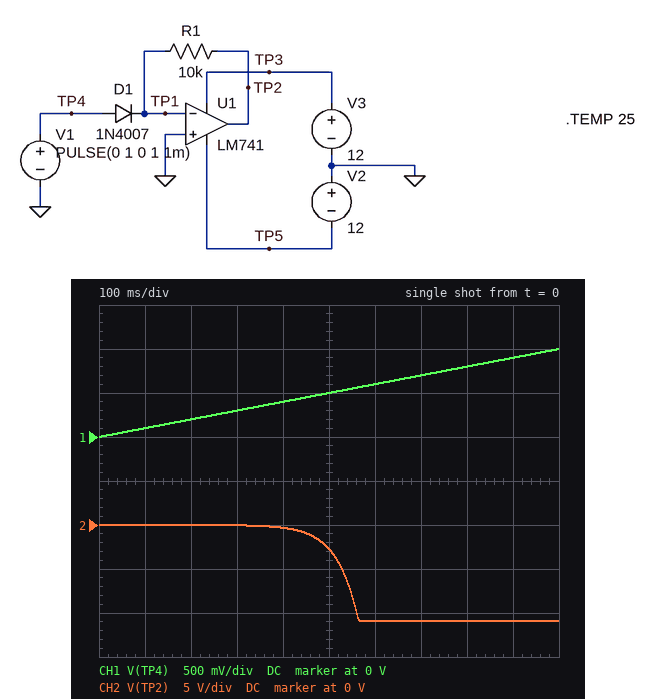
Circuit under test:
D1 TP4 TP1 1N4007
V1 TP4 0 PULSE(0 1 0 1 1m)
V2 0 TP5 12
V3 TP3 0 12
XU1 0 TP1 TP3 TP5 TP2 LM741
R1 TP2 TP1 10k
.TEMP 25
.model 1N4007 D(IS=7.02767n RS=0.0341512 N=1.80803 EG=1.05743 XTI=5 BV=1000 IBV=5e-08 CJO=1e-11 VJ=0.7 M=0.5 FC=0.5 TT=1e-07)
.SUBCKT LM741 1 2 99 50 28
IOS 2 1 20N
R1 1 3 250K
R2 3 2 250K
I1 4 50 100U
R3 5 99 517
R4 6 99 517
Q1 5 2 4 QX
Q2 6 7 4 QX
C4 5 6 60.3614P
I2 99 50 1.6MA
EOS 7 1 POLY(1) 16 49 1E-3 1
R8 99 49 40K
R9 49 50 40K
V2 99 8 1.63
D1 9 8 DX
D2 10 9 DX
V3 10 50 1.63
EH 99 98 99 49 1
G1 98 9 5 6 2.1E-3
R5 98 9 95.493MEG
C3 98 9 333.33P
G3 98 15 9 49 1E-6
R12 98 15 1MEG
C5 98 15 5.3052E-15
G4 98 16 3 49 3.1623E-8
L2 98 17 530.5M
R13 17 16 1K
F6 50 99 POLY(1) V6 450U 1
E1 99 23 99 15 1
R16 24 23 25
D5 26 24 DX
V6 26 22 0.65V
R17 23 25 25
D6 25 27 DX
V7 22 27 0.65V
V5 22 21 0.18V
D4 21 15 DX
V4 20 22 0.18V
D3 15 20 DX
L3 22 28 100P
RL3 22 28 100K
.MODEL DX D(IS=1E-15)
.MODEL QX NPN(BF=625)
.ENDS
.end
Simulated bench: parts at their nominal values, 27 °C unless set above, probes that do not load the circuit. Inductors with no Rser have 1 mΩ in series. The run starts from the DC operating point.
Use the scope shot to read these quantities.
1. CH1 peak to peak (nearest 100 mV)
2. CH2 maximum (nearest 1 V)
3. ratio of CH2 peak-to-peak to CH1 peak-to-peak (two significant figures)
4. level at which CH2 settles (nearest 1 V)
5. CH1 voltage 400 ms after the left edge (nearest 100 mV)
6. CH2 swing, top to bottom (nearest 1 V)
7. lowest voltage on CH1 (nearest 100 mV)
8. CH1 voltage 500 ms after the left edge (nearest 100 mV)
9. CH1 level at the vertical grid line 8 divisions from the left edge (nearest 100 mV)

1.0 V
0 V
11
-11 V
400 mV
11 V
0 V
500 mV
800 mV
